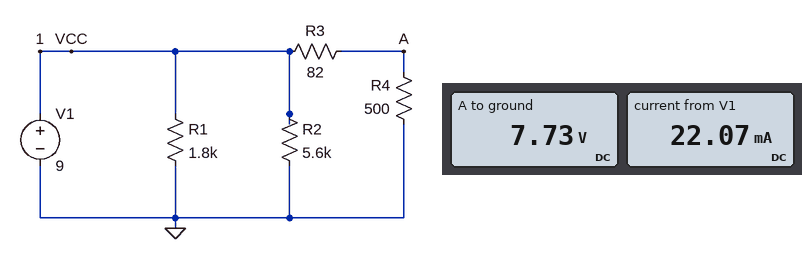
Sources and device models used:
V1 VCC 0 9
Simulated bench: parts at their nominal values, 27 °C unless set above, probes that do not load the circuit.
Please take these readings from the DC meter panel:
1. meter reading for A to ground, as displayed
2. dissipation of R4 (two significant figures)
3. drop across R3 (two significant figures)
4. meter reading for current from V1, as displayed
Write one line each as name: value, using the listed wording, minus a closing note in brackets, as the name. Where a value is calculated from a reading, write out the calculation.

meter reading for A to ground, as displayed: 7.73 V
dissipation of R4: (7.73 V)^2 / 500 Ω = 120 mW
drop across R3: 9 V - 7.73 V = 1.3 V
meter reading for current from V1, as displayed: 22.07 mA
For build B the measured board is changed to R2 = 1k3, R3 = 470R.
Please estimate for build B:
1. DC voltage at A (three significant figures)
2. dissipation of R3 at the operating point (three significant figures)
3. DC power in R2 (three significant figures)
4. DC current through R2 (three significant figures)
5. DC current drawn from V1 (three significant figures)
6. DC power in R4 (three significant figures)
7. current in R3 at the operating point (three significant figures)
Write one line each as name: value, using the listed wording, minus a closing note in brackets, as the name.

DC voltage at A: 4.64 V
dissipation of R3 at the operating point: 40.5 mW
DC power in R2: 62.3 mW
DC current through R2: 6.92 mA
DC current drawn from V1: 21.2 mA
DC power in R4: 43.0 mW
current in R3 at the operating point: 9.28 mA
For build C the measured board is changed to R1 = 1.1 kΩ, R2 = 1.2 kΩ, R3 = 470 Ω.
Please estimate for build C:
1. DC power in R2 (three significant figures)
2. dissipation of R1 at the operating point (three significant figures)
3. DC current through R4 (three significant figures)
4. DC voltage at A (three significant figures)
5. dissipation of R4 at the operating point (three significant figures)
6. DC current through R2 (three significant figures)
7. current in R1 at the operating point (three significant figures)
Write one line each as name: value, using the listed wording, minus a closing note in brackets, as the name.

DC power in R2: 67.5 mW
dissipation of R1 at the operating point: 73.6 mW
DC current through R4: 9.28 mA
DC voltage at A: 4.64 V
dissipation of R4 at the operating point: 43.0 mW
DC current through R2: 7.50 mA
current in R1 at the operating point: 8.18 mA
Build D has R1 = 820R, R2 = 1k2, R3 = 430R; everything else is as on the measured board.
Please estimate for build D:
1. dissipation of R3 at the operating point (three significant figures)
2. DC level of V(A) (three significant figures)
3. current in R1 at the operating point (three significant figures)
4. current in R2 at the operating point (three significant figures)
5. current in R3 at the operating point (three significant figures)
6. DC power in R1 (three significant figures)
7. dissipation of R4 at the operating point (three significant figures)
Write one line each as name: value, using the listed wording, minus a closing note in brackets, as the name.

dissipation of R3 at the operating point: 40.3 mW
DC level of V(A): 4.84 V
current in R1 at the operating point: 11.0 mA
current in R2 at the operating point: 7.50 mA
current in R3 at the operating point: 9.68 mA
DC power in R1: 98.8 mW
dissipation of R4 at the operating point: 46.8 mW
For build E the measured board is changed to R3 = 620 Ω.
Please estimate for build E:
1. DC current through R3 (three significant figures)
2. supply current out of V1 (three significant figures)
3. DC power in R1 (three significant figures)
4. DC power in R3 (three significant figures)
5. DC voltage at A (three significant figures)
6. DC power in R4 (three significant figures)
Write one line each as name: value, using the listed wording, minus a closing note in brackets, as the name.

DC current through R3: 8.04 mA
supply current out of V1: 14.6 mA
DC power in R1: 45.0 mW
DC power in R3: 40.0 mW
DC voltage at A: 4.02 V
DC power in R4: 32.3 mW
